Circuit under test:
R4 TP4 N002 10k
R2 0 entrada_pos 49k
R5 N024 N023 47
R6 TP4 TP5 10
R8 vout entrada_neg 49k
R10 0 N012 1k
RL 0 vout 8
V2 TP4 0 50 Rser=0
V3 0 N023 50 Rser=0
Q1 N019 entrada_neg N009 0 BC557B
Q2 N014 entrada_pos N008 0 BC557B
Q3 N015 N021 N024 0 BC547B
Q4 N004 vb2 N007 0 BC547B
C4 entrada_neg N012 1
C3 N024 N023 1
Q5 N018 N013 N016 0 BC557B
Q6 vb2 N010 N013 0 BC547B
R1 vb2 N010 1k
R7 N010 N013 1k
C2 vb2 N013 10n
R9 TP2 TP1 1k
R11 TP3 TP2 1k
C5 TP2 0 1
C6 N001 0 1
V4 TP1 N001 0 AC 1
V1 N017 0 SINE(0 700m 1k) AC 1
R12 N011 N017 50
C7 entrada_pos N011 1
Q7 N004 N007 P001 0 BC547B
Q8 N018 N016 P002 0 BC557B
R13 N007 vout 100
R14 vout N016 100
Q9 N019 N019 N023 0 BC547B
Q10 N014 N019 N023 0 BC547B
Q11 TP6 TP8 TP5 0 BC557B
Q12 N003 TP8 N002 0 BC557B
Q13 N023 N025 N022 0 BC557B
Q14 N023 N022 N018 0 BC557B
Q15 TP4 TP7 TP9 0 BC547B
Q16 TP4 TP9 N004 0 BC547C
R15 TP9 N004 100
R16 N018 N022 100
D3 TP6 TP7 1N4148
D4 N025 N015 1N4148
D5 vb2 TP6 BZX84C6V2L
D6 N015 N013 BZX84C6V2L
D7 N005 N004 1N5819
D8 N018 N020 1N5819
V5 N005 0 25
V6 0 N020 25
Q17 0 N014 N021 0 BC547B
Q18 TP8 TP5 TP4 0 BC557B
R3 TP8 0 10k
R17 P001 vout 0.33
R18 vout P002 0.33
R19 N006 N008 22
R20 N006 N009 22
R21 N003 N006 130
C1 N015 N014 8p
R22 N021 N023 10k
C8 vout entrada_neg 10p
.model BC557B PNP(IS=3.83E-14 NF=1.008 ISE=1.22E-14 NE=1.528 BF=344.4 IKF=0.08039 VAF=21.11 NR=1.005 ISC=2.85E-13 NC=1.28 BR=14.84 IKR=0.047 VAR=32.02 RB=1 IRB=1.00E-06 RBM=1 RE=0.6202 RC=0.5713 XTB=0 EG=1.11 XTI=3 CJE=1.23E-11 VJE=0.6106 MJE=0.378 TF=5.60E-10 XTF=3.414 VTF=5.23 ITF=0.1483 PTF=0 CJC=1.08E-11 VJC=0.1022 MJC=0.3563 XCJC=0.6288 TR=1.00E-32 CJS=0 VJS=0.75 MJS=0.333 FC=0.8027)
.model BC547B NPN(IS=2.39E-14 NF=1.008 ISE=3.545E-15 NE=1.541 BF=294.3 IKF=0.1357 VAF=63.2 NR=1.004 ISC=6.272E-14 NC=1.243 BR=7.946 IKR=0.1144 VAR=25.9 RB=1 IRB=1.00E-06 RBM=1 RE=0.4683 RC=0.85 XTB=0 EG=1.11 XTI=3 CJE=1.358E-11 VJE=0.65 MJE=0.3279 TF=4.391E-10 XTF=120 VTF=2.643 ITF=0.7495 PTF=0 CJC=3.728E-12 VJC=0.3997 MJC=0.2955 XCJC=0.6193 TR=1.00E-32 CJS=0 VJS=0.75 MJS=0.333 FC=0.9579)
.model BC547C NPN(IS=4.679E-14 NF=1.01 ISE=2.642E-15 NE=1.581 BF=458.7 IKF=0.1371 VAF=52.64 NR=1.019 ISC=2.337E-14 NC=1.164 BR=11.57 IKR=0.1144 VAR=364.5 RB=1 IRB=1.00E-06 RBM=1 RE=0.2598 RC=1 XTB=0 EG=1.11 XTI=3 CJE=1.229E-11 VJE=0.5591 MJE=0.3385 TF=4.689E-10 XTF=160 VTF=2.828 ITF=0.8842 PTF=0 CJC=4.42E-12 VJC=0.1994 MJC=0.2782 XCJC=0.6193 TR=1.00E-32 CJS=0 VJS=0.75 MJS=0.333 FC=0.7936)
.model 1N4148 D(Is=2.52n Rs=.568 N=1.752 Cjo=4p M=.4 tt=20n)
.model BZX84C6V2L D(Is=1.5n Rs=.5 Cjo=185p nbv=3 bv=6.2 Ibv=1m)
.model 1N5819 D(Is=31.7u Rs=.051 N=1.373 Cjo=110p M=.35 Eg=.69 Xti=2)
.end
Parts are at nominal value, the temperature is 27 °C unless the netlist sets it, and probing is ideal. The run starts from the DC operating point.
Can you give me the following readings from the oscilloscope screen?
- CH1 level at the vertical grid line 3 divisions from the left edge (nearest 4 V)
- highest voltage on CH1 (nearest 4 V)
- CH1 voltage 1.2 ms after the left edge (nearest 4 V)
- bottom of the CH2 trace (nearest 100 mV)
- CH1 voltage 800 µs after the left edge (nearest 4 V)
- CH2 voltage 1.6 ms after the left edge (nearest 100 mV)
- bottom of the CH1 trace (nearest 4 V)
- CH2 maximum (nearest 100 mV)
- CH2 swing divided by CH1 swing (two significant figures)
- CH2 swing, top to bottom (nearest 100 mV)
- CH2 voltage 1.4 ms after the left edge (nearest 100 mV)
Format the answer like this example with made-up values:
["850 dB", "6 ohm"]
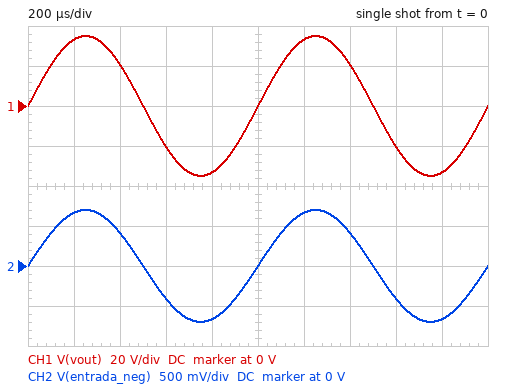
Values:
["-20 V", "36 V", "32 V", "-700 mV", "-32 V", "-400 mV", "-36 V", "700 mV", "0.020", "1.4 V", "400 mV"]
